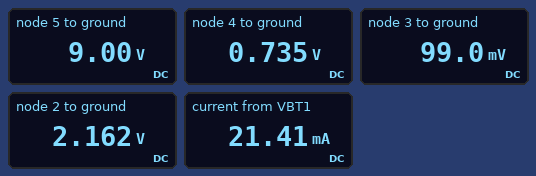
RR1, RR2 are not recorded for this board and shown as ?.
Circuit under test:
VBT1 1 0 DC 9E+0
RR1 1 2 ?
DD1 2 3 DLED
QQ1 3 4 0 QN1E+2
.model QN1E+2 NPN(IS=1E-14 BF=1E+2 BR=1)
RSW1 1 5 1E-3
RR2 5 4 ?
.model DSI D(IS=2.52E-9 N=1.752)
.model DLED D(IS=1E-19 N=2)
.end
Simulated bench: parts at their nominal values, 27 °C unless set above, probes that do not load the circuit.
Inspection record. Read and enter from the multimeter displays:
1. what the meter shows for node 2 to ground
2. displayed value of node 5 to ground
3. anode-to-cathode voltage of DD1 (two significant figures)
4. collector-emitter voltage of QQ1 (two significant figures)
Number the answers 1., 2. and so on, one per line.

1. 2.162 V
2. 9.00 V
3. 2.1 V
4. 99 mV
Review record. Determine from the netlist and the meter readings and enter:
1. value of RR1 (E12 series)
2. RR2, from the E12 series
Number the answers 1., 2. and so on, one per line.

1. 330 Ω
2. 12 kΩ
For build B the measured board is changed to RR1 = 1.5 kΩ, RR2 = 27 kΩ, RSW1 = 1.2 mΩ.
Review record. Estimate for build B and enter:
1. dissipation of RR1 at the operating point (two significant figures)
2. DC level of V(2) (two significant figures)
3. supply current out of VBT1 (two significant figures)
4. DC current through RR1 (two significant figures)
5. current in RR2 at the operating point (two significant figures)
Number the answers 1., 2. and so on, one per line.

1. 32 mW
2. 2.1 V
3. 4.9 mA
4. 4.6 mA
5. 310 µA
